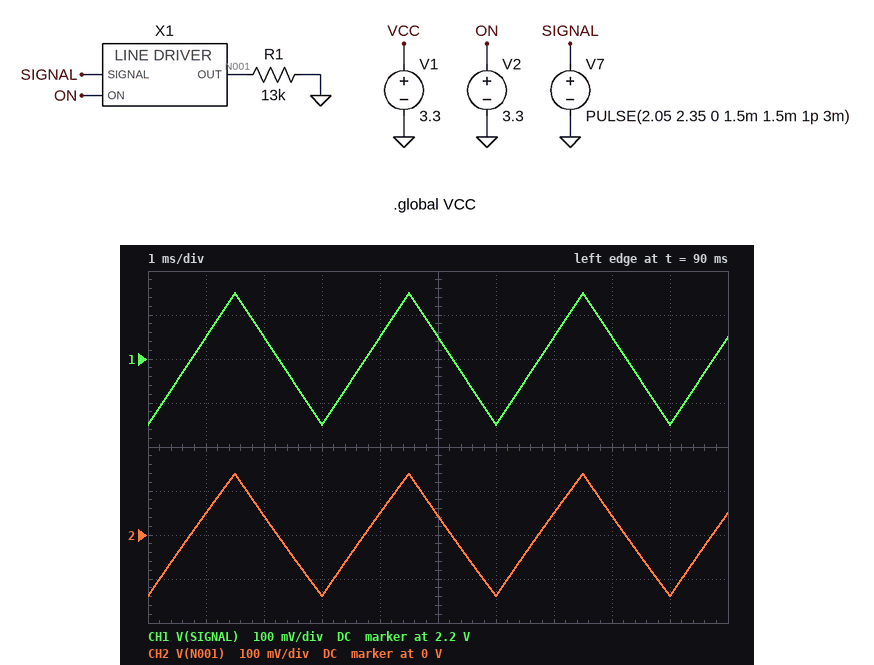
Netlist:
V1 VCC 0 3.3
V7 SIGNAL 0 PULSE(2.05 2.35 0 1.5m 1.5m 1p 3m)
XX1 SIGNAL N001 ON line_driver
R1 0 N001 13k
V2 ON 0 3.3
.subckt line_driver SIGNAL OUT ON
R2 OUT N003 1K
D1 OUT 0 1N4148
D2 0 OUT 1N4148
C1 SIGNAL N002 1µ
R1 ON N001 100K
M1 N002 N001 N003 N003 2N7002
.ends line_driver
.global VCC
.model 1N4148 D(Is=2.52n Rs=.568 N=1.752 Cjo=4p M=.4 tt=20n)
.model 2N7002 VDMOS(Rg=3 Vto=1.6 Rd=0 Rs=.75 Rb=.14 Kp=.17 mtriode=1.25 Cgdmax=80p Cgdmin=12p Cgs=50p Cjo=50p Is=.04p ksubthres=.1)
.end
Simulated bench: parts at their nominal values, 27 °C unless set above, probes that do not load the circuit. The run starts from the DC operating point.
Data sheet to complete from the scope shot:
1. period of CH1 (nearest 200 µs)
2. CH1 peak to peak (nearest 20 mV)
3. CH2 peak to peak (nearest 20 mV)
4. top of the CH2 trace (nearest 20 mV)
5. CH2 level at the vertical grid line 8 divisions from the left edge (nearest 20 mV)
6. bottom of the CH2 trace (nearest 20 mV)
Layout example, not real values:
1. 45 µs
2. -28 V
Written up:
1. 3.0 ms
2. 300 mV
3. 280 mV
4. 140 mV
5. 40 mV
6. -140 mV
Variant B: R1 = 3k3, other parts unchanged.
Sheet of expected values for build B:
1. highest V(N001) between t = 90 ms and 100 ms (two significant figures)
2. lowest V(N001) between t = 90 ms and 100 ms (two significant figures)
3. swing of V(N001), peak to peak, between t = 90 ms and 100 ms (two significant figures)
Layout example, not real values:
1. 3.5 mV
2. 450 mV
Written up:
1. 110 mV
2. -110 mV
3. 230 mV
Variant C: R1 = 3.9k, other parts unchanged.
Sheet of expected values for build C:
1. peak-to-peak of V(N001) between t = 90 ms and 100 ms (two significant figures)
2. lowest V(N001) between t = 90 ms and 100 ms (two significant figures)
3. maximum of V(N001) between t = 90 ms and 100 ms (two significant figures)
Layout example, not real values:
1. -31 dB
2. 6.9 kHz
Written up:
1. 240 mV
2. -120 mV
3. 120 mV
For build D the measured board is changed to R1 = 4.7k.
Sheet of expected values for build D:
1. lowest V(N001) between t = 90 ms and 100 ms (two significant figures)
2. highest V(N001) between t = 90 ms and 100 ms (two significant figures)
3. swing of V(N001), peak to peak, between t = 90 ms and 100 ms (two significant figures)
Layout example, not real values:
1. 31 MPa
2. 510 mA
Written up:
1. -120 mV
2. 120 mV
3. 250 mV
